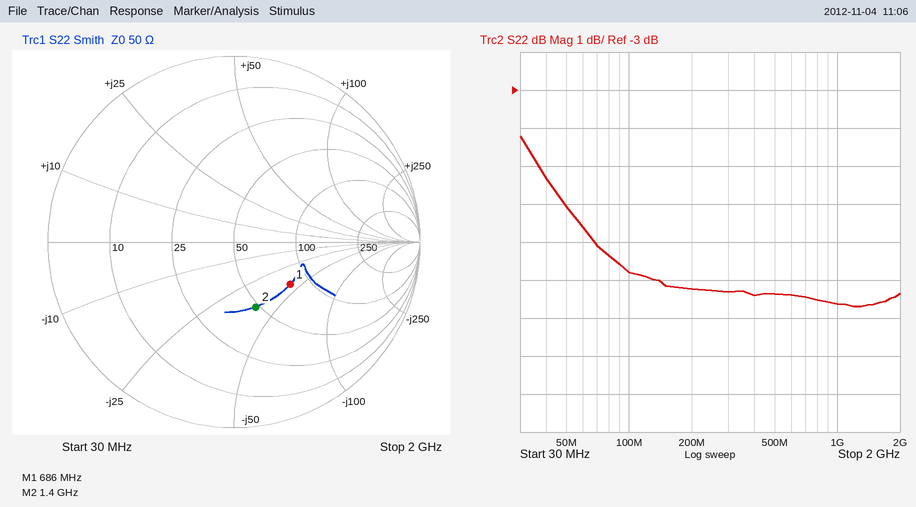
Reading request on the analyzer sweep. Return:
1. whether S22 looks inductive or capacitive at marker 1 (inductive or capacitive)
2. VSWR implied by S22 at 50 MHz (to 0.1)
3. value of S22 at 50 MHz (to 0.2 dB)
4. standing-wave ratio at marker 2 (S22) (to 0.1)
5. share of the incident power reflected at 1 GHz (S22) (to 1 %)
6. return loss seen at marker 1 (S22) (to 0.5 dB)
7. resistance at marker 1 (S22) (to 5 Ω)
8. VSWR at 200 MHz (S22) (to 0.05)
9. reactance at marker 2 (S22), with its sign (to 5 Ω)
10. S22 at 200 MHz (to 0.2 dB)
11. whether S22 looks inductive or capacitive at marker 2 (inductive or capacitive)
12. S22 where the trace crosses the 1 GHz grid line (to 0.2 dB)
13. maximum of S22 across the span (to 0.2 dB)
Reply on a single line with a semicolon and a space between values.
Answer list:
capacitive; 3.0; -6.0 dB; 2.2; 14 %; 8.5 dB; 80 Ω; 2.25; -40 Ω; -8.2 dB; capacitive; -8.6 dB; -4.2 dB
